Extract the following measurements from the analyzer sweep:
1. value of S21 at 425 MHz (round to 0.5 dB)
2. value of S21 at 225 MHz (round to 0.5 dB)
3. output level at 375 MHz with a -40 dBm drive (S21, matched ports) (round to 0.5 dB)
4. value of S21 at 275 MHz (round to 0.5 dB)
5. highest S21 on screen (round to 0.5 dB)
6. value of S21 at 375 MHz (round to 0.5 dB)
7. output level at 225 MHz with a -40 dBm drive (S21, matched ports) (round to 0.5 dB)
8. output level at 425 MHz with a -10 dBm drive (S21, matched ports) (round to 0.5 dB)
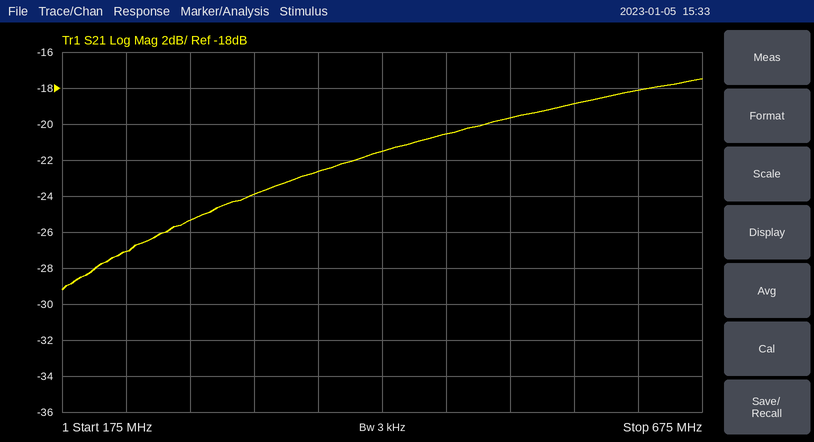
-21.5 dB
-27.0 dB
-62.5 dBm
-25.5 dB
-17.5 dB
-22.5 dB
-67.0 dBm
-31.5 dBm
